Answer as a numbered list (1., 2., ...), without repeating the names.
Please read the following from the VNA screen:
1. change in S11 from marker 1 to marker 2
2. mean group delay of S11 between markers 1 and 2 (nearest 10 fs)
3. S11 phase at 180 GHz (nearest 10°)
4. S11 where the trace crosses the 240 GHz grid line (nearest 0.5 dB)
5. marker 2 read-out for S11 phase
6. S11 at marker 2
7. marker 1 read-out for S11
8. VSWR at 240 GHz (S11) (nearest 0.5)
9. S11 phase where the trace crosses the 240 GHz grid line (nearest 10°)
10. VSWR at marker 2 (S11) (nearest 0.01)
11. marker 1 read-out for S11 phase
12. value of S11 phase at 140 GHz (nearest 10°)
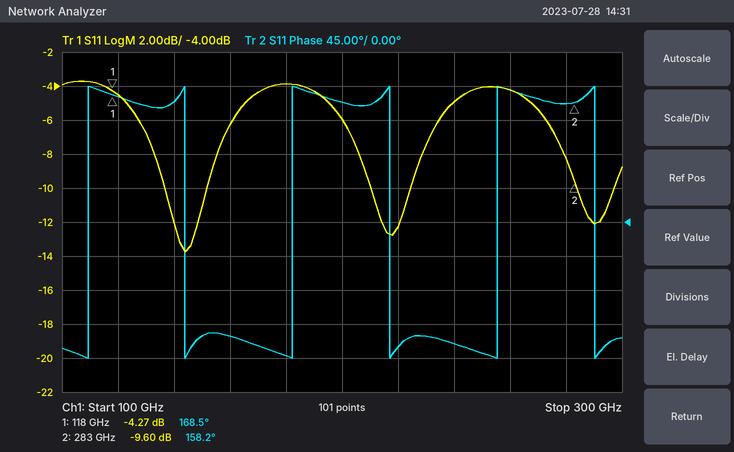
1. -5.33 dB
2. 170 fs
3. -180°
4. -5.0 dB
5. 158.2°
6. -9.60 dB
7. -4.27 dB
8. 3.5
9. -160°
10. 1.99
11. 168.5°
12. 160°
